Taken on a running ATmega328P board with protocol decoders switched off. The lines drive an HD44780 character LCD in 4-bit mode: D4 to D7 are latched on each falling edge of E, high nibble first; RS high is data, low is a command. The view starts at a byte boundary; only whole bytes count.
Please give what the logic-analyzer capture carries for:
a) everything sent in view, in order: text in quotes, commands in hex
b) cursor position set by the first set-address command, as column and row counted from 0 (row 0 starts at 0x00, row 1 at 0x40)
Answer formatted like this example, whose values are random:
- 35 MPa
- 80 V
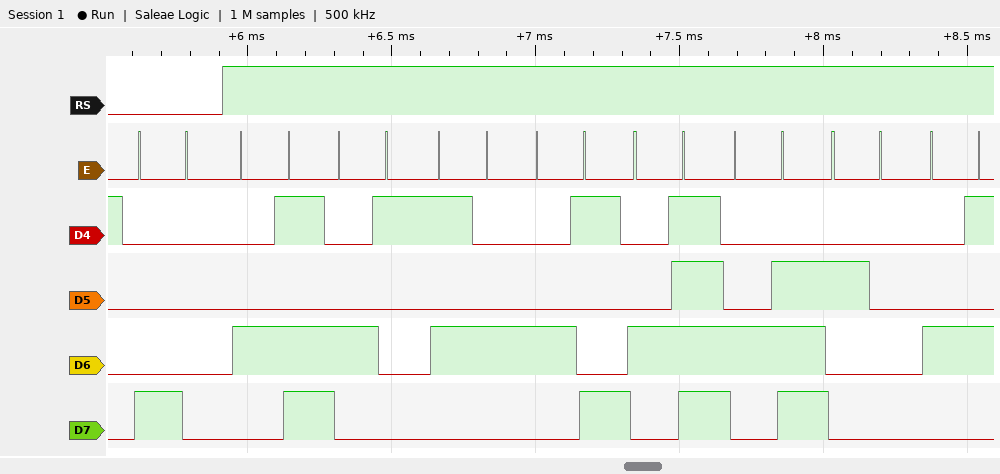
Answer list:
- 0x80 "MATION E"
- column 0, row 0
